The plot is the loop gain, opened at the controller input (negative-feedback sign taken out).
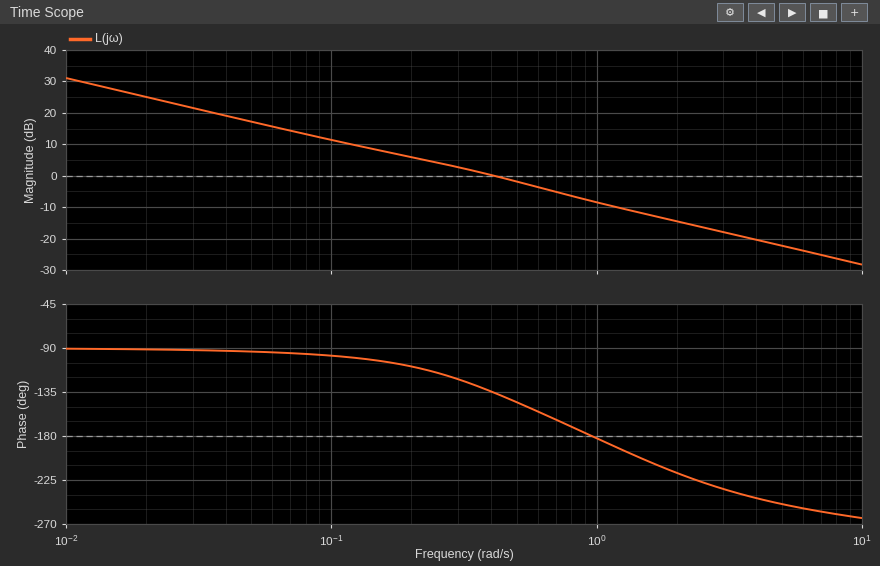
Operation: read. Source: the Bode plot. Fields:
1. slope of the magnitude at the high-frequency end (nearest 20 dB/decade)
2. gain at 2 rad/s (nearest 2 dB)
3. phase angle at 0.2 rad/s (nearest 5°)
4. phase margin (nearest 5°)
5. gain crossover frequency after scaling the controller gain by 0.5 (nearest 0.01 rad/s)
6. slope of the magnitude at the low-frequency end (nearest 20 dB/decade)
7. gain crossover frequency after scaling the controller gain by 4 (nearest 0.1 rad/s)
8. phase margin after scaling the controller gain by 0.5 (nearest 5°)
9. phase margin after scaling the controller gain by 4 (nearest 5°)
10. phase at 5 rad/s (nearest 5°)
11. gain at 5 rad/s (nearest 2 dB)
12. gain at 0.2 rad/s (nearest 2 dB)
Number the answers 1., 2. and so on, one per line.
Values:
1. -20 dB/decade
2. -14 dB
3. -110°
4. 45°
5. 0.20 rad/s
6. -20 dB/decade
7. 1.5 rad/s
8. 70°
9. -25°
10. -250°
11. -22 dB
12. 6 dB
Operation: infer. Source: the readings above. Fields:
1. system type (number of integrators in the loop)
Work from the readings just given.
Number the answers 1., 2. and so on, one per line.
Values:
1. 1
